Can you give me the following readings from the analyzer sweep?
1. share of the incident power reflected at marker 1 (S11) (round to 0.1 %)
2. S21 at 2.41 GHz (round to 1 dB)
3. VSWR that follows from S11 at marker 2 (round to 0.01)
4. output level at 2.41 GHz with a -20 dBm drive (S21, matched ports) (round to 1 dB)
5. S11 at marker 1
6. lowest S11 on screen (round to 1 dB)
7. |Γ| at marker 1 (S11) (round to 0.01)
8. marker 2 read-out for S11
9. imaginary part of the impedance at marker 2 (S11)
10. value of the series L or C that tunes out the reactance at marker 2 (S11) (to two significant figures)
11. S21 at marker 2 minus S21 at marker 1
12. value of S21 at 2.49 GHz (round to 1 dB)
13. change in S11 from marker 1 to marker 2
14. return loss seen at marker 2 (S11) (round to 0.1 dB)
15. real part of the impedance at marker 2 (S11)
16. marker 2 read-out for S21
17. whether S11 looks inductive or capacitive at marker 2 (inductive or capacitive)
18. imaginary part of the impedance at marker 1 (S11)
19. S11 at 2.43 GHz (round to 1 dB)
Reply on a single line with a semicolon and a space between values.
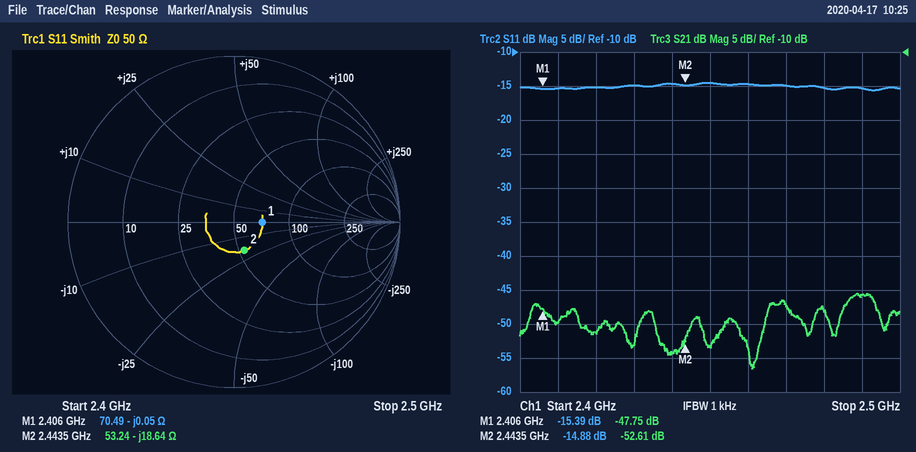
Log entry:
2.9 %; -50 dB; 1.44; -70 dBm; -15.39 dB; -16 dB; 0.17; -14.88 dB; -18.64 Ω; 1.2 nH; -4.86 dB; -46 dB; 0.51 dB; 14.9 dB; 53.24 Ω; -52.61 dB; capacitive; -0.05 Ω; -15 dB
